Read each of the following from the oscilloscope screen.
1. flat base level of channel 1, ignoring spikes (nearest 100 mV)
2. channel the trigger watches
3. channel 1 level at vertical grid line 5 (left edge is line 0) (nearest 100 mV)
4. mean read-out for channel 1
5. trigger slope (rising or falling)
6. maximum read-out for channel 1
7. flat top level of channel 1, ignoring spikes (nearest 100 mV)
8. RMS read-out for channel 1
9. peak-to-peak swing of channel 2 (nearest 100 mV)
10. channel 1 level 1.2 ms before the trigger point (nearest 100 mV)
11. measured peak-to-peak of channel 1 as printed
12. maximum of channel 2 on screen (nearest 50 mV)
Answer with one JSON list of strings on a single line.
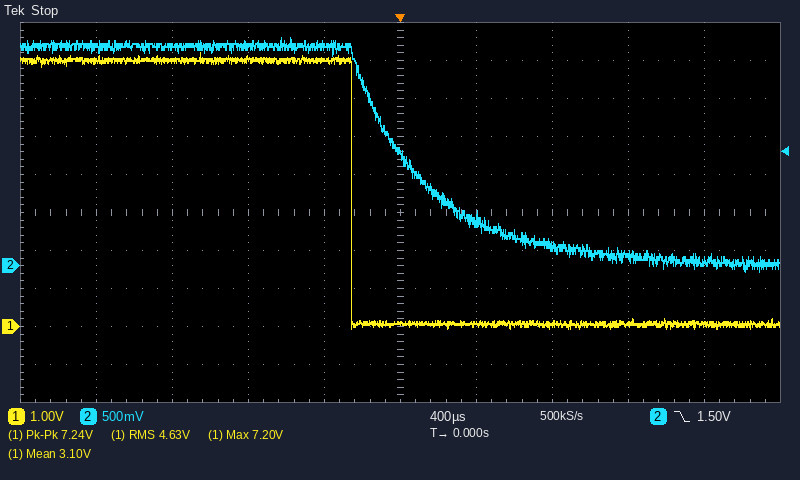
["100 mV", "channel 2", "100 mV", "3.10 V", "falling", "7.20 V", "7.0 V", "4.63 V", "3.10 V", "7.0 V", "7.24 V", "3.00 V"]
